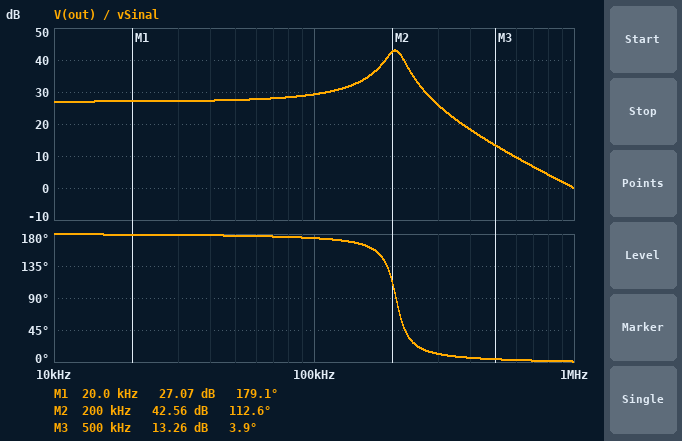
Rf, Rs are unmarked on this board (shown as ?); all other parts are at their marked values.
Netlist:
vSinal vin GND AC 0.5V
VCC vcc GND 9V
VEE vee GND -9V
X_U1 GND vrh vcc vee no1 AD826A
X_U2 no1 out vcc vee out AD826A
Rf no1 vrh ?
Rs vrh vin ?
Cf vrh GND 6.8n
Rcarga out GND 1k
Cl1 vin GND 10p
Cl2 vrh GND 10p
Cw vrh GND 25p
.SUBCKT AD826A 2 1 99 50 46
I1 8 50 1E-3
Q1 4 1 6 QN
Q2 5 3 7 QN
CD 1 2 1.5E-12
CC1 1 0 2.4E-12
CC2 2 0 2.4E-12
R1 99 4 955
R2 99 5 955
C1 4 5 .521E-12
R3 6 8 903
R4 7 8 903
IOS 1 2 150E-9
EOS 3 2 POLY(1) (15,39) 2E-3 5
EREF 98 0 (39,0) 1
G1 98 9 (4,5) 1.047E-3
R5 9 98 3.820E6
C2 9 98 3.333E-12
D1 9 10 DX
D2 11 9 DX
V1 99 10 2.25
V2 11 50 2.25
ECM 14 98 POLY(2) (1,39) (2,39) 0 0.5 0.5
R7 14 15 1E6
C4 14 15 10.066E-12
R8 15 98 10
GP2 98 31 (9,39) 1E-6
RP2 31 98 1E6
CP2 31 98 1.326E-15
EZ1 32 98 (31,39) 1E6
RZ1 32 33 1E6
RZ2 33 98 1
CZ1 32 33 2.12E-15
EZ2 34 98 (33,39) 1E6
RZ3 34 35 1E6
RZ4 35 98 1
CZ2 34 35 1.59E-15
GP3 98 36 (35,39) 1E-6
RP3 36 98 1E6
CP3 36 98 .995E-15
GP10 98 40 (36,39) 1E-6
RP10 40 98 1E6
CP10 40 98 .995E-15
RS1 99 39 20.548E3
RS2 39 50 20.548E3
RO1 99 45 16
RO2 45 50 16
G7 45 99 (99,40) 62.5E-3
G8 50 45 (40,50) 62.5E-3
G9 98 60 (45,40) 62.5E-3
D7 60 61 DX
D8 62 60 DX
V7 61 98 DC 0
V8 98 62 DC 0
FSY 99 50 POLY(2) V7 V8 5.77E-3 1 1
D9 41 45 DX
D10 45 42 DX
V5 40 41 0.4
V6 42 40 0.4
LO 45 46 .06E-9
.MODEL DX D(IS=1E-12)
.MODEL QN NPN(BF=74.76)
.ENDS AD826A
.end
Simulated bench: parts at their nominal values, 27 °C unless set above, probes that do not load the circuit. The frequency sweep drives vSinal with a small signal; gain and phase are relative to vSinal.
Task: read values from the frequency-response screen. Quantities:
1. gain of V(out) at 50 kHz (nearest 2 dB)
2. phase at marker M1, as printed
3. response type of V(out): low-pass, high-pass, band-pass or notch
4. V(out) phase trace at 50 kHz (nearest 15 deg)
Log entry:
28 dB
179.1 deg
low-pass
180 deg
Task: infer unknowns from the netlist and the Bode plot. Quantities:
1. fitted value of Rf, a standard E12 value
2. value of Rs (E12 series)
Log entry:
27 kΩ
1.2 kΩ
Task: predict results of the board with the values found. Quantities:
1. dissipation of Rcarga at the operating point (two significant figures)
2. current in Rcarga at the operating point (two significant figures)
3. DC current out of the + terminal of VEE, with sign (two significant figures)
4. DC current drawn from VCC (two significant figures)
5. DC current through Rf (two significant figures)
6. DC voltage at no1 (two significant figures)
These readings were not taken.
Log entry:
53 µW
230 µA
-14 mA
15 mA
8.4 µA
230 mV
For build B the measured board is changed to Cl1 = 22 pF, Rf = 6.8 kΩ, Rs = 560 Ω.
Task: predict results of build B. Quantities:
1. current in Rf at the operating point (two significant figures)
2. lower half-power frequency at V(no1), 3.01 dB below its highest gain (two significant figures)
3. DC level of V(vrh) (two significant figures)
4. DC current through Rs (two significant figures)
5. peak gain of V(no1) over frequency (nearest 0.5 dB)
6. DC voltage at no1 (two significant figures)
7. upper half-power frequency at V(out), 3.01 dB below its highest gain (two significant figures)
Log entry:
10 µA
380 kHz
2.0 mV
3.5 µA
39.0 dB
72 mV
440 kHz
